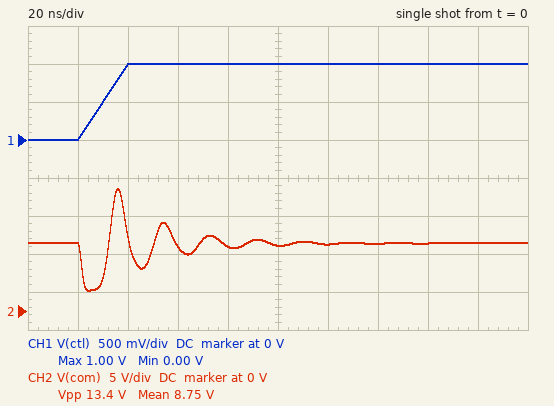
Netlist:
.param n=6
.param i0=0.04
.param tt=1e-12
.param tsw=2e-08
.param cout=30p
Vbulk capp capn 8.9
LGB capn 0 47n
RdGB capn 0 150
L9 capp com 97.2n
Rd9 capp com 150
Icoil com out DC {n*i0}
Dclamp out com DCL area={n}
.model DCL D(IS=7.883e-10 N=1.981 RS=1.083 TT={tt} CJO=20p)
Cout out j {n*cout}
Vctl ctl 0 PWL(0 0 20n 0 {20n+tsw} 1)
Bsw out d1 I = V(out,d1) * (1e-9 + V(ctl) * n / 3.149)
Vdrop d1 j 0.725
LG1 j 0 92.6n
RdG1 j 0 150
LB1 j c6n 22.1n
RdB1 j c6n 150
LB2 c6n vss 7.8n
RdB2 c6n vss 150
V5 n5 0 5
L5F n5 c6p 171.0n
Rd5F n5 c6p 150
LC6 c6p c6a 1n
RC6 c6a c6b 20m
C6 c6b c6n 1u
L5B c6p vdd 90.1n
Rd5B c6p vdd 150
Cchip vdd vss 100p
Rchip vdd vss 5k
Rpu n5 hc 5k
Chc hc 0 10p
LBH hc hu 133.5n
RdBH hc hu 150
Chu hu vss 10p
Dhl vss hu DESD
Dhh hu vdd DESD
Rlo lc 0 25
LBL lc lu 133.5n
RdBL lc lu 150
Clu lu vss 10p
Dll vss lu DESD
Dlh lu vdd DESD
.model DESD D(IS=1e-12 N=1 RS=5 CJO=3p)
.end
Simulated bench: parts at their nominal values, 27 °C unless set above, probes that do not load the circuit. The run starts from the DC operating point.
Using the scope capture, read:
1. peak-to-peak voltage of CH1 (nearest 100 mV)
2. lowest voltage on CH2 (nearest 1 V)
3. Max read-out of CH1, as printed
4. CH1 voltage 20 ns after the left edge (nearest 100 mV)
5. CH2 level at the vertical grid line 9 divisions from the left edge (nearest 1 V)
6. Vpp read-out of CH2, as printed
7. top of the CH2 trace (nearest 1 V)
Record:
1.0 V
3 V
1.00 V
0 V
9 V
13.4 V
16 V
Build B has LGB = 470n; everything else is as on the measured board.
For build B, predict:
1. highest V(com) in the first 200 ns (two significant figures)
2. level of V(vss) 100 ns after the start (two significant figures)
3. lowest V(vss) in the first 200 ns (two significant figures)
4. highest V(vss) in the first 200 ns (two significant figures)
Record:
15 V
60 mV
-860 mV
1.0 V
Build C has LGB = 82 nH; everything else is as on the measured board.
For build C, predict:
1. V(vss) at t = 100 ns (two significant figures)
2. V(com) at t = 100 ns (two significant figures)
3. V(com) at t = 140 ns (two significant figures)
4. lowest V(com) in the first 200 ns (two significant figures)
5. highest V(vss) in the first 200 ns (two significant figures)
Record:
-200 mV
9.4 V
9.0 V
2.3 V
1.8 V
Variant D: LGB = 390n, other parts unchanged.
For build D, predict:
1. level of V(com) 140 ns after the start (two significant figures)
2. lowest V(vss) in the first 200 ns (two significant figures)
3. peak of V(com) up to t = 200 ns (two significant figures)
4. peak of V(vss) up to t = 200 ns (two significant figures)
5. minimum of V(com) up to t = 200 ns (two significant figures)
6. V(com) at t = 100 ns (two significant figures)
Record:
9.0 V
-1.0 V
15 V
1.1 V
1.0 V
8.5 V
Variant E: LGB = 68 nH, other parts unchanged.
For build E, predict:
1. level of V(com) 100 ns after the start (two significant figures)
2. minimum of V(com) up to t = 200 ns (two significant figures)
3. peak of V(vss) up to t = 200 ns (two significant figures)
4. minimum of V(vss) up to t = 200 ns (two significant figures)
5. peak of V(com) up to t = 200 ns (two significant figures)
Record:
9.0 V
2.4 V
1.9 V
-2.3 V
16 V
